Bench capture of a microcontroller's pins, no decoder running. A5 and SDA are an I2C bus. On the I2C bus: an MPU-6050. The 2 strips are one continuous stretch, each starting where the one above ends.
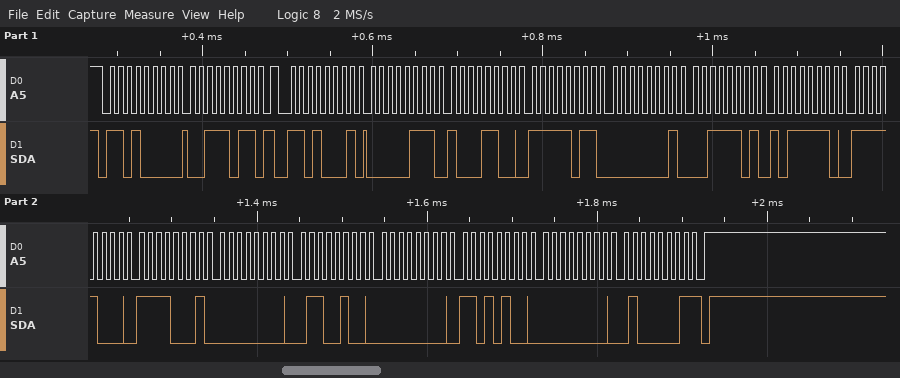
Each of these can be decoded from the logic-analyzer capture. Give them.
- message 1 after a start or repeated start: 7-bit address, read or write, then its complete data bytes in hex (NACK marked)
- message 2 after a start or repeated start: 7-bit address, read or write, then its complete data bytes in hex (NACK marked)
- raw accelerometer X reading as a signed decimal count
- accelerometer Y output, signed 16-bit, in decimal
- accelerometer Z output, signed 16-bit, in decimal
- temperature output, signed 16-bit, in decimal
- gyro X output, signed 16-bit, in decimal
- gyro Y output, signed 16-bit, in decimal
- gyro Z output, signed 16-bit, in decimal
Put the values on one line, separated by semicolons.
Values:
0x68 write: 3B; 0x68 read: 07 8C FB 01 3D BE F8 F1 00 64 00 D4 00 41 NACK; 1932; -1279; 15806; -1807; 100; 212; 65
